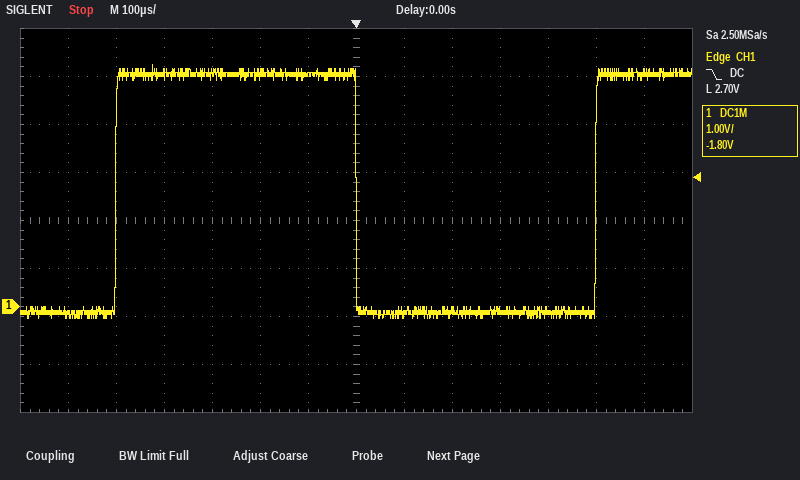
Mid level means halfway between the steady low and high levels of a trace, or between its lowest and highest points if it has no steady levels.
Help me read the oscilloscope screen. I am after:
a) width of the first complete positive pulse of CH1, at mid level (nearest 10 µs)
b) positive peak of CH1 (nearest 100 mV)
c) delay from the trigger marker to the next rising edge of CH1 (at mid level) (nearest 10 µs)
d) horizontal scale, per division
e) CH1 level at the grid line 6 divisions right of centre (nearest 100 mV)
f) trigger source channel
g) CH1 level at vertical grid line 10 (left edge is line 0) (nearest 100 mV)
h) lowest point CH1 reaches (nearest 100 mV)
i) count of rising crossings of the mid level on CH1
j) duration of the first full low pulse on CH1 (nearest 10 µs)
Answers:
500 µs
5.0 V
500 µs
100 µs
4.9 V
CH1
-100 mV
-200 mV
2
500 µs
